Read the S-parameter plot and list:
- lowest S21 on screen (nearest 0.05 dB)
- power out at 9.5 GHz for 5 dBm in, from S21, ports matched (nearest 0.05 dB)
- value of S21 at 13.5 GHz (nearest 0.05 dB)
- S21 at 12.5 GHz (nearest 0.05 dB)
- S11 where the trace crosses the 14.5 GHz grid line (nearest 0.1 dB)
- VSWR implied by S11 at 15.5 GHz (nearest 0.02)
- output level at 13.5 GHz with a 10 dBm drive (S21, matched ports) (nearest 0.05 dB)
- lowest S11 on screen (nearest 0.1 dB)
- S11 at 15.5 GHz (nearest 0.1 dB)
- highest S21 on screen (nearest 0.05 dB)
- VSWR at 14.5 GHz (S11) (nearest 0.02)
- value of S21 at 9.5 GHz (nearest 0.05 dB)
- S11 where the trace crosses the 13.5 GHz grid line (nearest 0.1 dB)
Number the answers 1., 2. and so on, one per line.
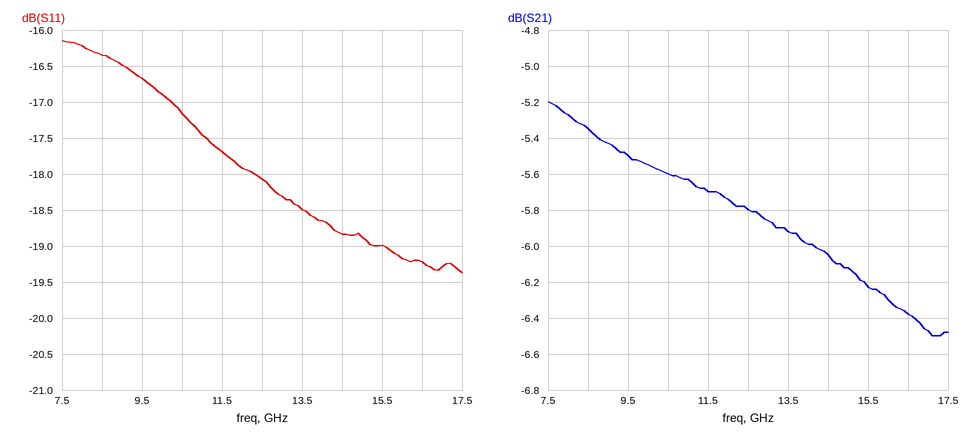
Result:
1. -6.50 dB
2. -0.50 dBm
3. -5.90 dB
4. -5.80 dB
5. -18.8 dB
6. 1.26
7. 4.10 dBm
8. -19.4 dB
9. -19.0 dB
10. -5.20 dB
11. 1.26
12. -5.50 dB
13. -18.5 dB
